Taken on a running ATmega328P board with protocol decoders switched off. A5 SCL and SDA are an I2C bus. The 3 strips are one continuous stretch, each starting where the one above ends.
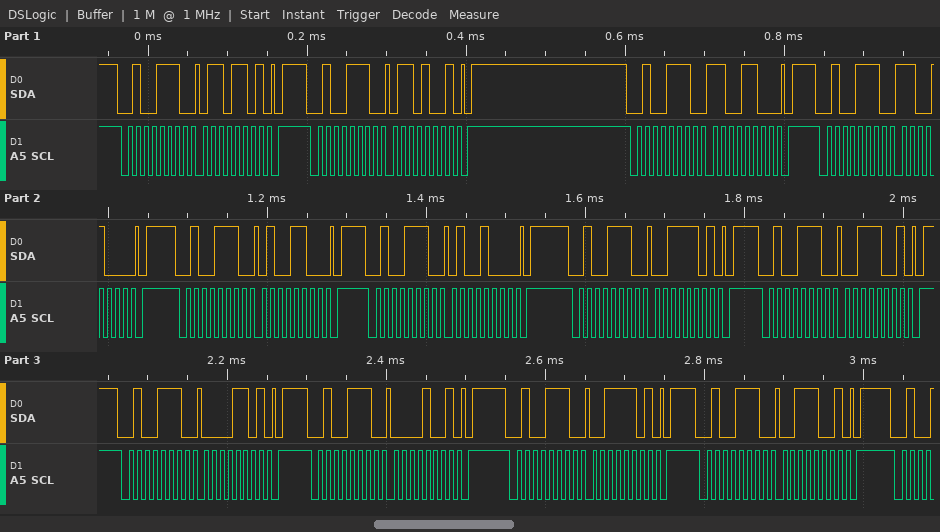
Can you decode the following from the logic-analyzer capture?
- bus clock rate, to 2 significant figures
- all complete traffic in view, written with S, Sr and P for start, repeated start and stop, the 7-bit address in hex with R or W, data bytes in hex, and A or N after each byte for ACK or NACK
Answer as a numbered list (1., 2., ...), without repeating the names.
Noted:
1. 100 kHz
2. S 27W A 6D A P S 27W A 69 A P S 27W A CC A P S 27W A C8 A P S 27W A 4C A P S 27W A 48 A P S 27W A 3D A P S 27W A 39 A P S 27W A 0D A P S 27W A 09 A P S 27W A 3D A P S 27W A 39 A P
